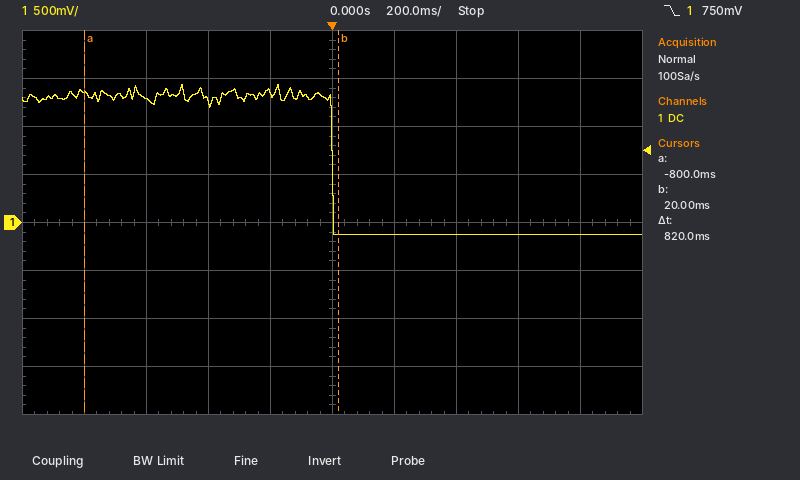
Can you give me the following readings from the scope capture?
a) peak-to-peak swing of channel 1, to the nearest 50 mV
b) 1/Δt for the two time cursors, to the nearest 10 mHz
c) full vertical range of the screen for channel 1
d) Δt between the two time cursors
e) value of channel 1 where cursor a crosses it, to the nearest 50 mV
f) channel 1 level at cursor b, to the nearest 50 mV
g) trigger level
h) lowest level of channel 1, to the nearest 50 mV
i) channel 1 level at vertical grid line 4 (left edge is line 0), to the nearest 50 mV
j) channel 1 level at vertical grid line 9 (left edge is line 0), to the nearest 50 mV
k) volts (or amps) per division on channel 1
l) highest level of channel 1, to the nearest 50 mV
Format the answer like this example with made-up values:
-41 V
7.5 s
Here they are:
1.55 V
1.22 Hz
4 V
820 ms
1.35 V
-100 mV
750 mV
-100 mV
1.35 V
-100 mV
500 mV
1.45 V
